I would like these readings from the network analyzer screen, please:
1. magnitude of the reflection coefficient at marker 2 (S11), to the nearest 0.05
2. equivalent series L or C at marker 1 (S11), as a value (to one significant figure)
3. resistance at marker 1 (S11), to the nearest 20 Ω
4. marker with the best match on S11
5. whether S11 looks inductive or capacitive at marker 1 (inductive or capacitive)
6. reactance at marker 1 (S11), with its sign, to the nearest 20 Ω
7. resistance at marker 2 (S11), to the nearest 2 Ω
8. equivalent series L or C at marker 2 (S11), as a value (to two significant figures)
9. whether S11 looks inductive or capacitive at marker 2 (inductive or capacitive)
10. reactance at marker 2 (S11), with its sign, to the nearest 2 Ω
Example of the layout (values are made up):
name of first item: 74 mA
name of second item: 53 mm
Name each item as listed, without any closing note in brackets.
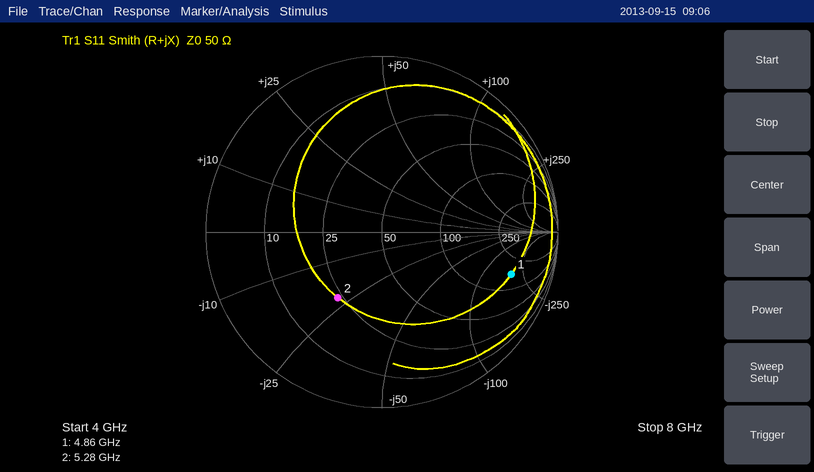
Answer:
magnitude of the reflection coefficient at marker 2 (S11), to the nearest 0.05: 0.45
equivalent series L or C at marker 1 (S11), as a value: 200 fF
resistance at marker 1 (S11), to the nearest 20 Ω: 160 Ω
marker with the best match on S11: marker 2
whether S11 looks inductive or capacitive at marker 1: capacitive
reactance at marker 1 (S11), with its sign, to the nearest 20 Ω: -180 Ω
resistance at marker 2 (S11), to the nearest 2 Ω: 24 Ω
equivalent series L or C at marker 2 (S11), as a value: 1.4 pF
whether S11 looks inductive or capacitive at marker 2: capacitive
reactance at marker 2 (S11), with its sign, to the nearest 2 Ω: -22 Ω
